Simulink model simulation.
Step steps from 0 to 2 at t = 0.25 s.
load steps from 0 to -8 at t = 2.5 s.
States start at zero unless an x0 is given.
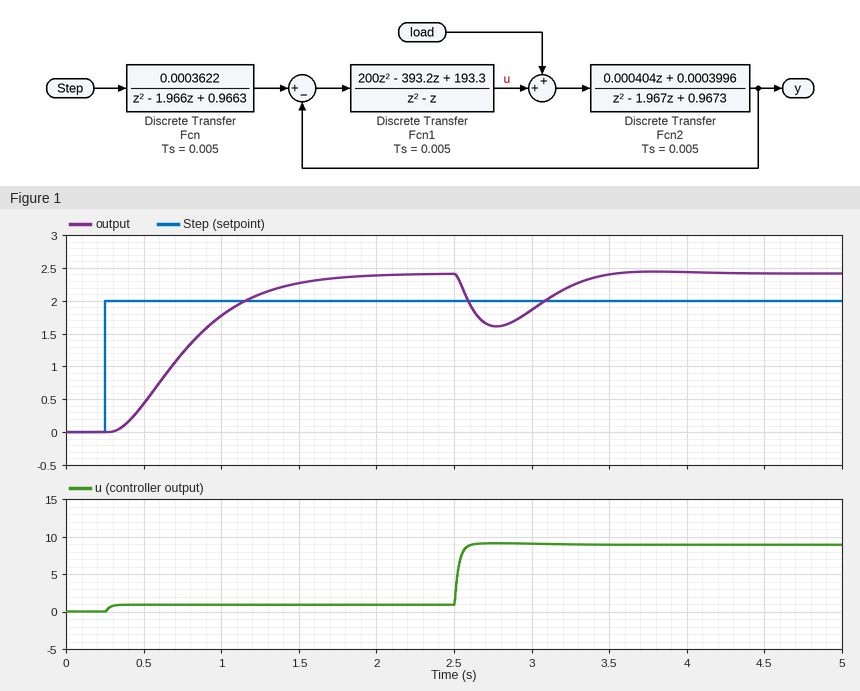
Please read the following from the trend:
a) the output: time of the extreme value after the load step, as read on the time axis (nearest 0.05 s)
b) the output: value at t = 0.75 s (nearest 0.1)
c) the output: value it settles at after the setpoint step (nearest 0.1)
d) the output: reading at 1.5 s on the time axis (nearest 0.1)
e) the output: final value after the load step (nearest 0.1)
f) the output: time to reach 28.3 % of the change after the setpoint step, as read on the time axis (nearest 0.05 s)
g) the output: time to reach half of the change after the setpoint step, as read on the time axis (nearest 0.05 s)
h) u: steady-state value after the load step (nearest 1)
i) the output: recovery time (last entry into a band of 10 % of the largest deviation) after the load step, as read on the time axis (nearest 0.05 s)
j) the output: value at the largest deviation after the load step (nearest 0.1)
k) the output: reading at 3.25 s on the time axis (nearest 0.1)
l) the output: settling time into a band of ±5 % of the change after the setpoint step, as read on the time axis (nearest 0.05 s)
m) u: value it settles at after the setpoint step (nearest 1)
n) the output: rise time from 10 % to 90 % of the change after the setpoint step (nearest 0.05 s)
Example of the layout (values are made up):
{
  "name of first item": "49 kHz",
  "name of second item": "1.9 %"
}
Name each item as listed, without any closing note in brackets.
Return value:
{
  "the output: time of the extreme value after the load step, as read on the time axis": "2.75 s",
  "the output: value at t = 0.75 s": "1.2",
  "the output: value it settles at after the setpoint step": "2.4",
  "the output: reading at 1.5 s on the time axis": "2.3",
  "the output: final value after the load step": "2.4",
  "the output: time to reach 28.3 % of the change after the setpoint step, as read on the time axis": "0.60 s",
  "the output: time to reach half of the change after the setpoint step, as read on the time axis": "0.75 s",
  "u: steady-state value after the load step": "9",
  "the output: recovery time (last entry into a band of 10 % of the largest deviation) after the load step, as read on the time axis": "3.40 s",
  "the output: value at the largest deviation after the load step": "1.6",
  "the output: reading at 3.25 s on the time axis": "2.2",
  "the output: settling time into a band of ±5 % of the change after the setpoint step, as read on the time axis": "1.55 s",
  "u: value it settles at after the setpoint step": "1",
  "the output: rise time from 10 % to 90 % of the change after the setpoint step": "0.90 s"
}
